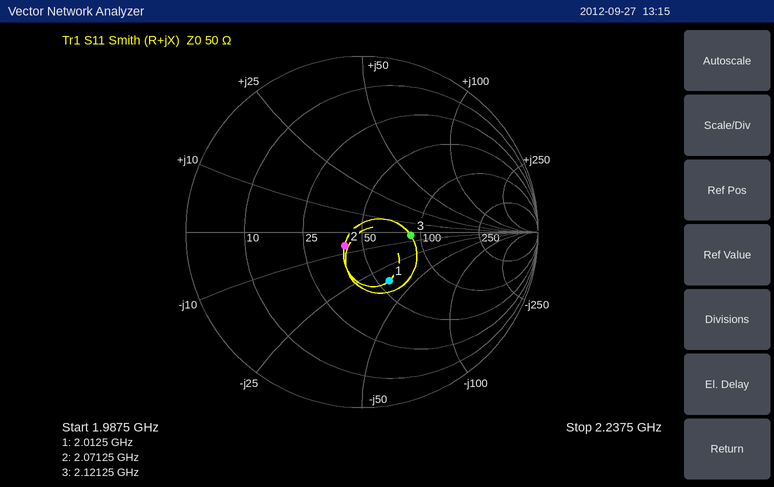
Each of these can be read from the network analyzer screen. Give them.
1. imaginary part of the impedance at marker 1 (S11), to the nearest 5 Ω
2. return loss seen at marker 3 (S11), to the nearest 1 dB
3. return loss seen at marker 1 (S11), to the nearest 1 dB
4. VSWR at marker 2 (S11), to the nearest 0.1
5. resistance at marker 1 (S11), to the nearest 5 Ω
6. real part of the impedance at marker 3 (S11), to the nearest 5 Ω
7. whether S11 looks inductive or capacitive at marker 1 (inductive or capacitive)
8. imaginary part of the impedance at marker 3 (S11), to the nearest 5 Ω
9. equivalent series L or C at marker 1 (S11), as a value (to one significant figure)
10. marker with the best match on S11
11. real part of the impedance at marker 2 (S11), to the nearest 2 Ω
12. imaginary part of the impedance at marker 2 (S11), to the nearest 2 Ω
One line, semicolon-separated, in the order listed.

-35 Ω; 11 dB; 10 dB; 1.3; 55 Ω; 90 Ω; capacitive; -5 Ω; 2 pF; marker 2; 40 Ω; -6 Ω
